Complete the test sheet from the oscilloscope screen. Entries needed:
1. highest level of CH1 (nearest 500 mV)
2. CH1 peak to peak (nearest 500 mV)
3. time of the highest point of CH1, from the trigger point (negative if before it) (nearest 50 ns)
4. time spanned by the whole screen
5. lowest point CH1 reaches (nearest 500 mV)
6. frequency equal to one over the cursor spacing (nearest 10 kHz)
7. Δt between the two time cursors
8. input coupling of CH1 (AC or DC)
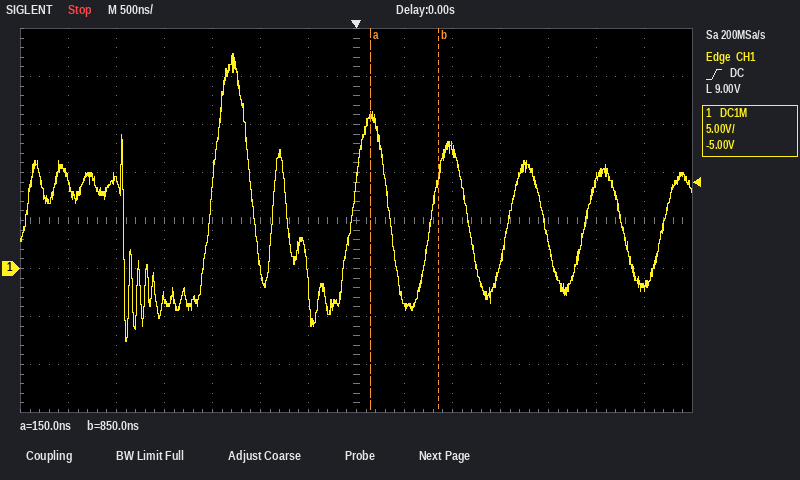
22.5 V
30.0 V
-1.30 µs
7 µs
-7.5 V
1.43 MHz
700 ns
DC
